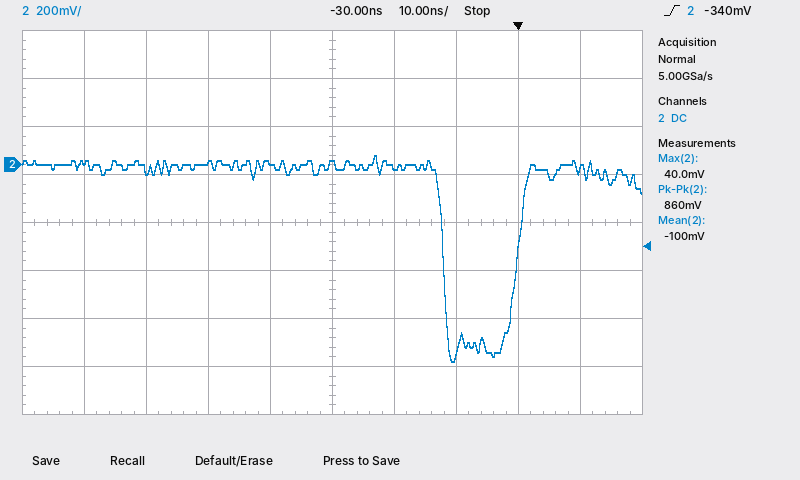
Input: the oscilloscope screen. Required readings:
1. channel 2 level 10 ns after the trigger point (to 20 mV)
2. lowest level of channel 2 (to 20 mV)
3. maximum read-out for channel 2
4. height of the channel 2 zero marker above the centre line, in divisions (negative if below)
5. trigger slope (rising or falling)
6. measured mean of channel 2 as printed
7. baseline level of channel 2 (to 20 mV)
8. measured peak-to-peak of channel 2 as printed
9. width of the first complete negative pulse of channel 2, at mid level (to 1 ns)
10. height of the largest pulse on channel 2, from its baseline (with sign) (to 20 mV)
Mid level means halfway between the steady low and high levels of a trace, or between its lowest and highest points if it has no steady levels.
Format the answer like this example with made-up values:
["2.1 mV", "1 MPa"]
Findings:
["-20 mV", "-820 mV", "40.0 mV", "+1.2 div", "rising", "-100 mV", "0 mV", "860 mV", "12 ns", "-820 mV"]
